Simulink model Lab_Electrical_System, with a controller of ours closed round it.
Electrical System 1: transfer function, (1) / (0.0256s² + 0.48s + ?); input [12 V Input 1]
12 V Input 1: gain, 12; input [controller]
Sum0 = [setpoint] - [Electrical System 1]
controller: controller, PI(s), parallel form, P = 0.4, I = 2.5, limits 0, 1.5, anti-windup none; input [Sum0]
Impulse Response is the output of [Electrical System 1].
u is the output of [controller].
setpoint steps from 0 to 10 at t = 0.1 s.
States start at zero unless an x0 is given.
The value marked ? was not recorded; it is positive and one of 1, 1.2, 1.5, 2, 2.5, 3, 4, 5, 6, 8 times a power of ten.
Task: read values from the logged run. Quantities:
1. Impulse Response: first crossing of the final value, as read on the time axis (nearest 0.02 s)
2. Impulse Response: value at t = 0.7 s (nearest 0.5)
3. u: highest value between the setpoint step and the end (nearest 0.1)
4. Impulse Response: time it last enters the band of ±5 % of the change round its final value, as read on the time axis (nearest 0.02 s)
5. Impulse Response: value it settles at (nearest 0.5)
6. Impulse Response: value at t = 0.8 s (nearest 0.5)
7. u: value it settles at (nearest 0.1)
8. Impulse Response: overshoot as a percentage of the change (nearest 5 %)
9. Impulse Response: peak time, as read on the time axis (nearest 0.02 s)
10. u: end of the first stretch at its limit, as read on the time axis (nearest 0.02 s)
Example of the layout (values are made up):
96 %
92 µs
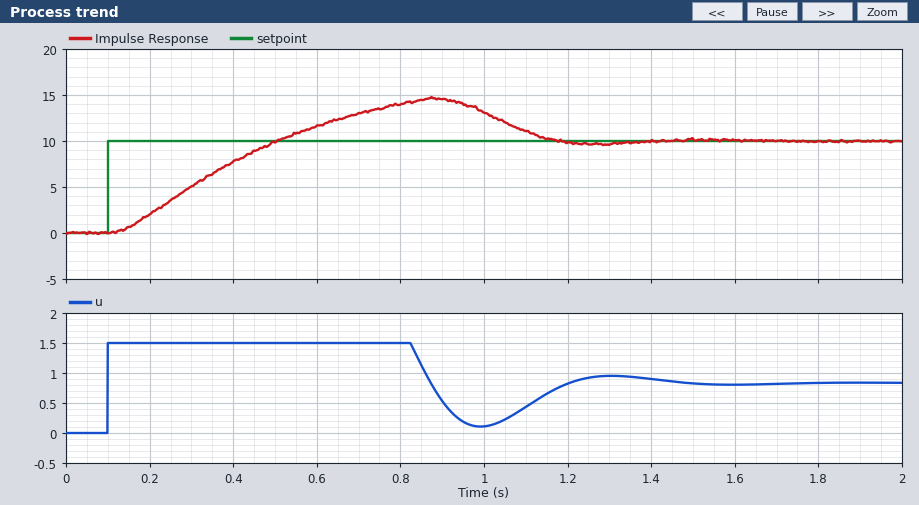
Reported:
0.50 s
13.0
1.5
1.14 s
10.0
14.0
0.8
45 %
0.88 s
0.82 s
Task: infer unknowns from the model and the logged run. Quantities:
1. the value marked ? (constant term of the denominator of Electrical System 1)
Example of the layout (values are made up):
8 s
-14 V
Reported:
1
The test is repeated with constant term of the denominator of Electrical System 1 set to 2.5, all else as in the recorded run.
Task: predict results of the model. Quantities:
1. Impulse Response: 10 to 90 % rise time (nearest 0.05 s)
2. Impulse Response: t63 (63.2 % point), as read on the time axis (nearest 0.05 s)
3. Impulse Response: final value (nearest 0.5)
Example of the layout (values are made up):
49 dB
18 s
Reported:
0.30 s
0.30 s
7.0
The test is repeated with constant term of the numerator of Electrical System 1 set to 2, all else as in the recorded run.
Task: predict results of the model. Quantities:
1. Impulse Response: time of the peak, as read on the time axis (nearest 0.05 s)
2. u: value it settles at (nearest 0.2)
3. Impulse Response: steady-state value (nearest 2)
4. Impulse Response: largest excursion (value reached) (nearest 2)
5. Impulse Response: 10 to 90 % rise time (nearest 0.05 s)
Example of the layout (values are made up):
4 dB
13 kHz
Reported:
0.45 s
0.4
10
16
0.15 s
